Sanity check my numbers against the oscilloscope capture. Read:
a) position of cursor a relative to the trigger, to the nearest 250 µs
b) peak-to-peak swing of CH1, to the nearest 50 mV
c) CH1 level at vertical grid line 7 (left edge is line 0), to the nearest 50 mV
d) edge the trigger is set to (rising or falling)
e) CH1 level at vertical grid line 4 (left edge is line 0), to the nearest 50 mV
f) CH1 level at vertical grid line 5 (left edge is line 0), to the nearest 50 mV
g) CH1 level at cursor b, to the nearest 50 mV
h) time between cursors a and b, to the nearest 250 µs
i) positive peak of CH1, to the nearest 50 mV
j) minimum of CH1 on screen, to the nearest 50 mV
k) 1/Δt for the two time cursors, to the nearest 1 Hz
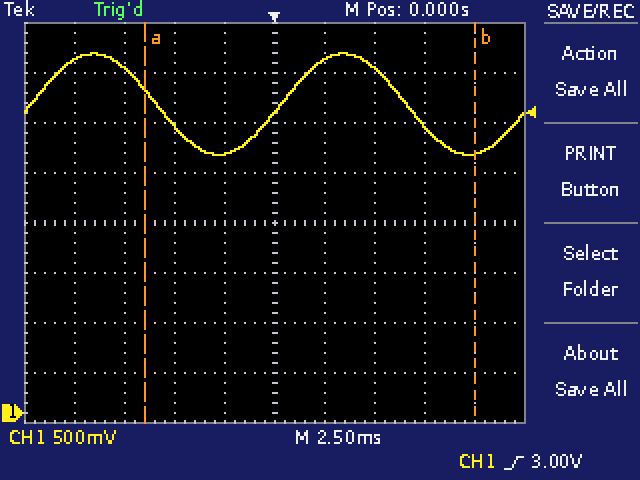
-6.50 ms
1.00 V
3.45 V
rising
2.60 V
3.00 V
2.60 V
16.50 ms
3.60 V
2.60 V
61 Hz
